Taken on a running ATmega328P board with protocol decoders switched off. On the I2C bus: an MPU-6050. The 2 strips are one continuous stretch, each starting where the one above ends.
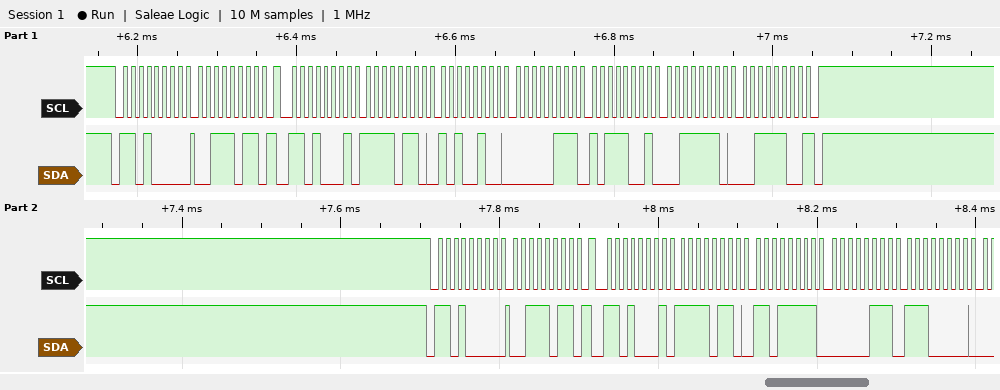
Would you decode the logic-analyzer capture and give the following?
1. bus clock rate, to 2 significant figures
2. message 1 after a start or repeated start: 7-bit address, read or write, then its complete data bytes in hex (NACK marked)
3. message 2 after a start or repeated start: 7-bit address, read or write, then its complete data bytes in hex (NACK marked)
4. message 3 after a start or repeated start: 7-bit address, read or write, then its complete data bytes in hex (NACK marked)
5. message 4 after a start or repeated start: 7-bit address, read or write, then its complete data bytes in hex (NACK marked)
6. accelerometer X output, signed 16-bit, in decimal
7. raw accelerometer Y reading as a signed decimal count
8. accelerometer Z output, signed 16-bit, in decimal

100 kHz
0x68 write: 3B
0x68 read: F6 A4 07 B9 3E 3C NACK
0x68 write: 3B
0x68 read: F6 DF 07 E0
-2396
1977
15932
